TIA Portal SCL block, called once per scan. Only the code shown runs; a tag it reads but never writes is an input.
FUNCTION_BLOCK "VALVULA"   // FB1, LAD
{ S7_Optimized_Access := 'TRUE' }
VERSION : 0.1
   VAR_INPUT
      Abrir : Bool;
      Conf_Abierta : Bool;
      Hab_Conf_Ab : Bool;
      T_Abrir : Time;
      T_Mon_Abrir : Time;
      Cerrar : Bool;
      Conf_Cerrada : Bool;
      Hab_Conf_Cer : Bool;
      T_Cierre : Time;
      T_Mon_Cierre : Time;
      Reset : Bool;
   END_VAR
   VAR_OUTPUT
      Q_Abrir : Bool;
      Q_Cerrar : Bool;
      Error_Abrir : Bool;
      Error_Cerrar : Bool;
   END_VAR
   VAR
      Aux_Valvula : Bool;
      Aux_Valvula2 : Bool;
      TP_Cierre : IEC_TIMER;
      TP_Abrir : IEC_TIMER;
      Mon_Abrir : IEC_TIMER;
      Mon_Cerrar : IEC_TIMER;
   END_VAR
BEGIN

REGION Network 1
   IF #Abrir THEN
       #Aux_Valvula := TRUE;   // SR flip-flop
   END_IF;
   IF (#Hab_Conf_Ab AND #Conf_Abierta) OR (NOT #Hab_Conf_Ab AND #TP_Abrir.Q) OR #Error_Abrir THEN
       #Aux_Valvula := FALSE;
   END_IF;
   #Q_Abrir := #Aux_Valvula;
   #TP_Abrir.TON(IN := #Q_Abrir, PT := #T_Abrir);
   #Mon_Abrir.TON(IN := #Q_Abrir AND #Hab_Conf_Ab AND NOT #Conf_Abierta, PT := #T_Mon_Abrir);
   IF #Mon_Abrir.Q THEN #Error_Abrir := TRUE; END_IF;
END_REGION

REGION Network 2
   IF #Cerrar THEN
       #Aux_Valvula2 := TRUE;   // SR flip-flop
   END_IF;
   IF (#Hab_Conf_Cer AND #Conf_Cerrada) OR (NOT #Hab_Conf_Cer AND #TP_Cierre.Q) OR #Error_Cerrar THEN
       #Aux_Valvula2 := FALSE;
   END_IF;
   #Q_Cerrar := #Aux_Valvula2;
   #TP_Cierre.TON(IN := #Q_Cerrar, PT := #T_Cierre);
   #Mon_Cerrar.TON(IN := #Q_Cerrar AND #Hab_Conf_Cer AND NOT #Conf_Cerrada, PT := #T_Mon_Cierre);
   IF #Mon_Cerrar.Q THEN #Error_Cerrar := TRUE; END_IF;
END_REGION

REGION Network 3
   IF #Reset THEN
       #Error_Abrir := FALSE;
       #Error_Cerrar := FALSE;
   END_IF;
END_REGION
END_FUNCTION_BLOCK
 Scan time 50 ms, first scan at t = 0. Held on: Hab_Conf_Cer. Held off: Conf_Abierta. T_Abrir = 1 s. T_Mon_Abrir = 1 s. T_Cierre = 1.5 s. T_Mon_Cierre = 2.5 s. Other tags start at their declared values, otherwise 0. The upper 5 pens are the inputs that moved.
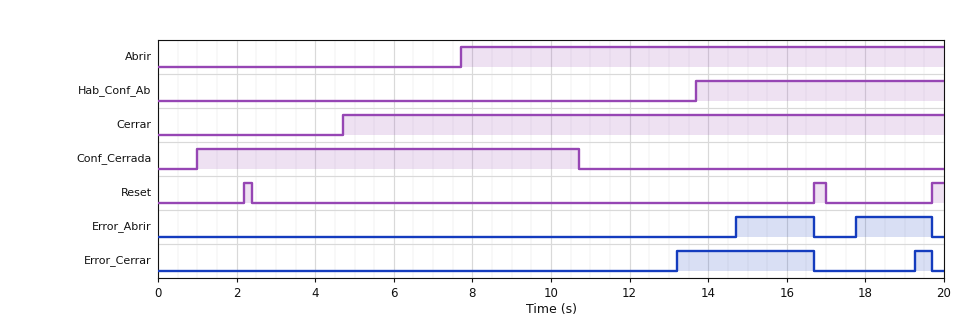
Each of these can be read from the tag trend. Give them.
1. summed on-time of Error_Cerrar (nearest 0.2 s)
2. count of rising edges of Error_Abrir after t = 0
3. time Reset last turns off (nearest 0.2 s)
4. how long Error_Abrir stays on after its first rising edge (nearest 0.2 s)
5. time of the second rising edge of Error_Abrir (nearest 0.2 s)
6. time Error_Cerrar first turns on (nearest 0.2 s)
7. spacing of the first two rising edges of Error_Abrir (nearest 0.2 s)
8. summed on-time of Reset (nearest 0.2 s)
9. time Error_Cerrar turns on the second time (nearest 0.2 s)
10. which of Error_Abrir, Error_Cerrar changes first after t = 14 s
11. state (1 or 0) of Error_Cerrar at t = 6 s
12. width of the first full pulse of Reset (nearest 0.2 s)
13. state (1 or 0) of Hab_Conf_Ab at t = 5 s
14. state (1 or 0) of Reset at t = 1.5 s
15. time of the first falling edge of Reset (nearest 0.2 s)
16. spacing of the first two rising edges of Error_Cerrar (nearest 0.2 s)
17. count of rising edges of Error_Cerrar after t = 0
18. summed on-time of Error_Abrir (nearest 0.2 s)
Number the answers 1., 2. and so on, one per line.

1. 4.0 s
2. 2
3. 17.0 s
4. 2.0 s
5. 17.8 s
6. 13.2 s
7. 3.0 s
8. 0.8 s
9. 19.2 s
10. Error_Abrir
11. 0
12. 0.2 s
13. 0
14. 0
15. 2.4 s
16. 6.0 s
17. 2
18. 4.0 s
